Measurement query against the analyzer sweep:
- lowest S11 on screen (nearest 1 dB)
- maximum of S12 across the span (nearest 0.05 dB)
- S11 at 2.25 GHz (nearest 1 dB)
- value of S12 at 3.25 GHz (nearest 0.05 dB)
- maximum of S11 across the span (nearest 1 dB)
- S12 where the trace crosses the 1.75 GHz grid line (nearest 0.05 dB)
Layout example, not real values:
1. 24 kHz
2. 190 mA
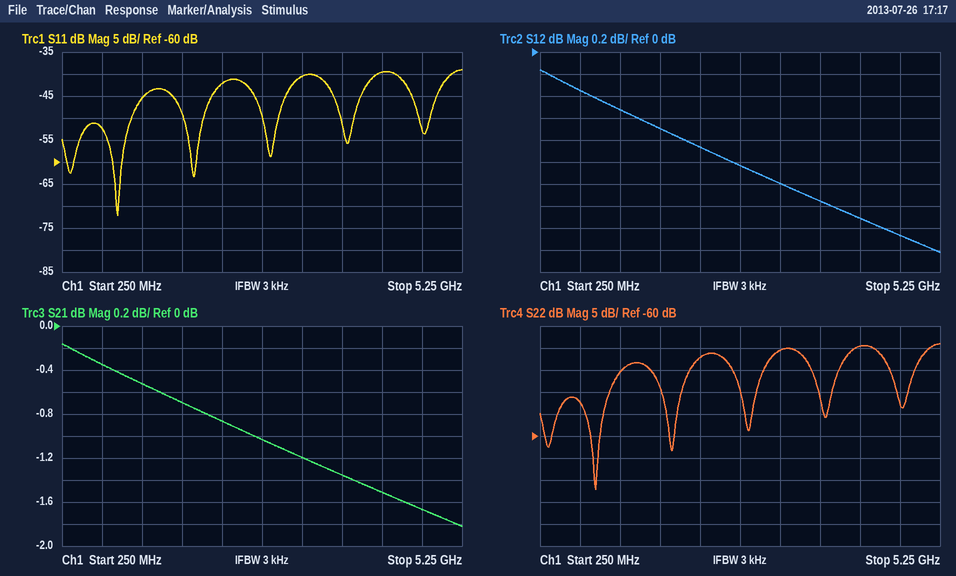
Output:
1. -72 dB
2. -0.15 dB
3. -42 dB
4. -1.20 dB
5. -39 dB
6. -0.70 dB
